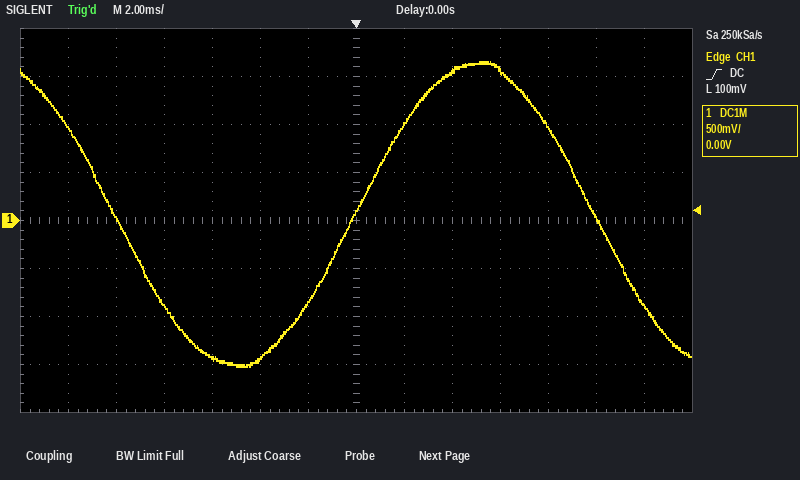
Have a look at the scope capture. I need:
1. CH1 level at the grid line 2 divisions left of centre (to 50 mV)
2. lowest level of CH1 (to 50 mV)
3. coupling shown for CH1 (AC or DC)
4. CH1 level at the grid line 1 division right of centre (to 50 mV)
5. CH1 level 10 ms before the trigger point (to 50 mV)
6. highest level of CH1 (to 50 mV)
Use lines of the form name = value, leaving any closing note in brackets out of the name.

CH1 level at the grid line 2 divisions left of centre = -1.45 V
lowest level of CH1 = -1.50 V
coupling shown for CH1 = DC
CH1 level at the grid line 1 division right of centre = 1.00 V
CH1 level 10 ms before the trigger point = 50 mV
highest level of CH1 = 1.65 V
